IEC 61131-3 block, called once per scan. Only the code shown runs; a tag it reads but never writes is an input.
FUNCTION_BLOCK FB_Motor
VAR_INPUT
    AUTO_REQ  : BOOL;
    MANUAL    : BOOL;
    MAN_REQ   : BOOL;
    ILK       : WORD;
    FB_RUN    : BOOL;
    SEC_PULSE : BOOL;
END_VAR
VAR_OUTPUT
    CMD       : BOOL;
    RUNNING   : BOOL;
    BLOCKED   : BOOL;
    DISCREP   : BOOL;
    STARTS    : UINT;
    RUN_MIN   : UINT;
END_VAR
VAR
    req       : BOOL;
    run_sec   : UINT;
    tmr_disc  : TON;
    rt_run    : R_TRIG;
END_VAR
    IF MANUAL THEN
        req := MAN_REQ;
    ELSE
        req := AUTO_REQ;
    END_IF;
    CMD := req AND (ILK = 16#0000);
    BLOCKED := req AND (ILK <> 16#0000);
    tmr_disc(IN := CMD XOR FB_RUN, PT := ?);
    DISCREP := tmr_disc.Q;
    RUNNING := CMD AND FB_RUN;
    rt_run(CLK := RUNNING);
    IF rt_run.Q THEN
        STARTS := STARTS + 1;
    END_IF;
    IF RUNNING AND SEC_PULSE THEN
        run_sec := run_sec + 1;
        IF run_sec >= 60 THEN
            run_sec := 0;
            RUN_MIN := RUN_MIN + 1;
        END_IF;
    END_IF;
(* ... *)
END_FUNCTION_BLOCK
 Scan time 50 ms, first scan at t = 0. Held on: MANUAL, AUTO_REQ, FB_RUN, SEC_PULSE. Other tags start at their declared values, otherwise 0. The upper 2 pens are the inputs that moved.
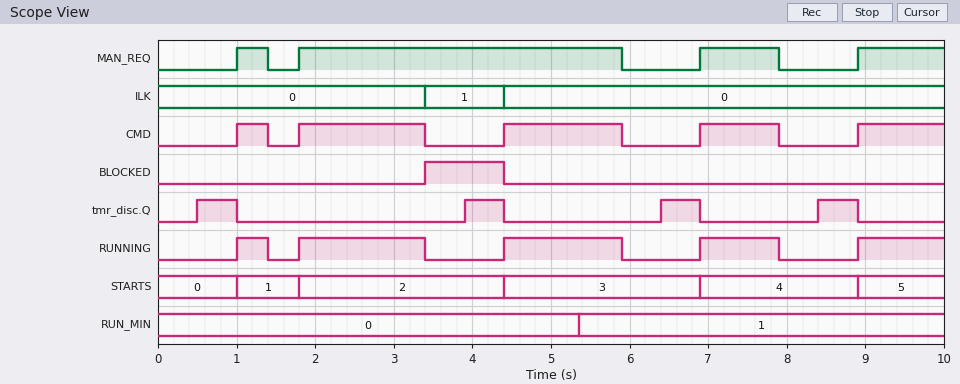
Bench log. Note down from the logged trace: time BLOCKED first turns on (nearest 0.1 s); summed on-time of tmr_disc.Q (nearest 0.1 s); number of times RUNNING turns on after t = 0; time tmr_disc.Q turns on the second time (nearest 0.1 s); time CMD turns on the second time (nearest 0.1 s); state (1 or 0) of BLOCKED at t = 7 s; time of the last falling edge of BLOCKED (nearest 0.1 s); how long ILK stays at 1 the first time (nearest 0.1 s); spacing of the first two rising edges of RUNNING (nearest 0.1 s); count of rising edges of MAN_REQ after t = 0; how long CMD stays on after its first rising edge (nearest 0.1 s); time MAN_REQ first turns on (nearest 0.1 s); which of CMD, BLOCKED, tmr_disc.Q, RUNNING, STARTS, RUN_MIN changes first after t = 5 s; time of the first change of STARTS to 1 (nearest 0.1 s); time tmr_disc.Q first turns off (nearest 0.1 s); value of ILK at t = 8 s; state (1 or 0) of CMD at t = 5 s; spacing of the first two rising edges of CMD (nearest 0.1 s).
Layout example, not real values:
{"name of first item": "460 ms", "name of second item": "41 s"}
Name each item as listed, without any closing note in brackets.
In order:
{"time BLOCKED first turns on": "3.4 s", "summed on-time of tmr_disc.Q": "2.0 s", "number of times RUNNING turns on after t = 0": "5", "time tmr_disc.Q turns on the second time": "3.9 s", "time CMD turns on the second time": "1.8 s", "state (1 or 0) of BLOCKED at t = 7 s": "0", "time of the last falling edge of BLOCKED": "4.4 s", "how long ILK stays at 1 the first time": "1.0 s", "spacing of the first two rising edges of RUNNING": "0.8 s", "count of rising edges of MAN_REQ after t = 0": "4", "how long CMD stays on after its first rising edge": "0.4 s", "time MAN_REQ first turns on": "1.0 s", "which of CMD, BLOCKED, tmr_disc.Q, RUNNING, STARTS, RUN_MIN changes first after t = 5 s": "RUN_MIN", "time of the first change of STARTS to 1": "1.0 s", "time tmr_disc.Q first turns off": "1.0 s", "value of ILK at t = 8 s": "0", "state (1 or 0) of CMD at t = 5 s": "1", "spacing of the first two rising edges of CMD": "0.8 s"}
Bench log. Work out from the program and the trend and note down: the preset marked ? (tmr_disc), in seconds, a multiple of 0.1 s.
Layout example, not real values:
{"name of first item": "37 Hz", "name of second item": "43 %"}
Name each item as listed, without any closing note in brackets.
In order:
{"the preset marked ? (tmr_disc), in seconds, a multiple of 0.1 s": "0.5 s"}
